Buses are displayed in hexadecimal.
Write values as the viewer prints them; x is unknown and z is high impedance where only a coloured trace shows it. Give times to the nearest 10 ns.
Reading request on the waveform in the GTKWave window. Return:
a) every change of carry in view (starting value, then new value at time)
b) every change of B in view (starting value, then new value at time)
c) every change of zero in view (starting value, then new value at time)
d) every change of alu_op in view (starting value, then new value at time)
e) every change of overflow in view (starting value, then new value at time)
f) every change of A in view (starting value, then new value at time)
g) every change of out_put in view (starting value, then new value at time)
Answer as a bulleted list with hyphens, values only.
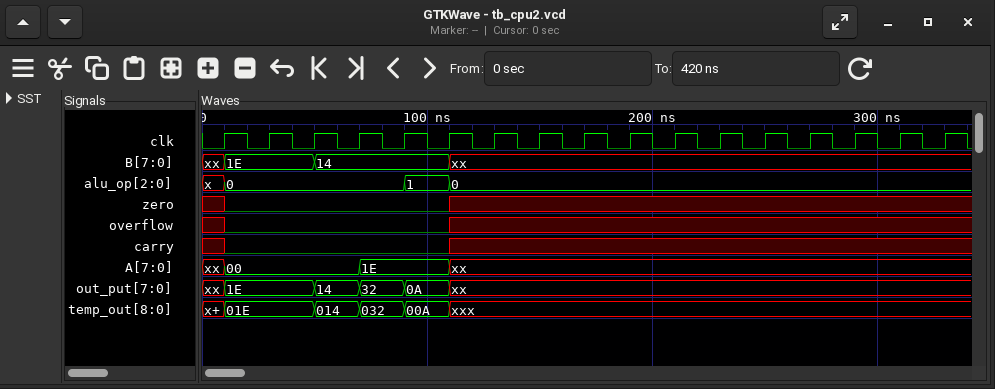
- x, 0 at 10 ns, x at 110 ns
- xx, 1E at 10 ns, 14 at 50 ns, xx at 110 ns
- x, 0 at 10 ns, x at 110 ns
- x, 0 at 10 ns, 1 at 90 ns, 0 at 110 ns
- x, 0 at 10 ns, x at 110 ns
- xx, 00 at 10 ns, 1E at 70 ns, xx at 110 ns
- xx, 1E at 10 ns, 14 at 50 ns, 32 at 70 ns, 0A at 90 ns, xx at 110 ns
